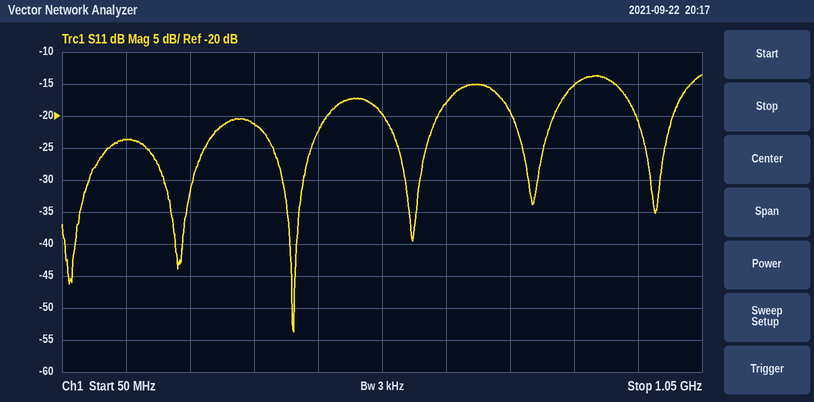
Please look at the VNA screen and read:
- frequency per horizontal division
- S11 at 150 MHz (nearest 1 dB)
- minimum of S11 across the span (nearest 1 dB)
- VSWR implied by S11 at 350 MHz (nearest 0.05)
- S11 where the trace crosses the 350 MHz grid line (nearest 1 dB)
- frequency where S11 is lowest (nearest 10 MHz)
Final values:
100 MHz
-24 dB
-54 dB
1.20
-21 dB
410 MHz
